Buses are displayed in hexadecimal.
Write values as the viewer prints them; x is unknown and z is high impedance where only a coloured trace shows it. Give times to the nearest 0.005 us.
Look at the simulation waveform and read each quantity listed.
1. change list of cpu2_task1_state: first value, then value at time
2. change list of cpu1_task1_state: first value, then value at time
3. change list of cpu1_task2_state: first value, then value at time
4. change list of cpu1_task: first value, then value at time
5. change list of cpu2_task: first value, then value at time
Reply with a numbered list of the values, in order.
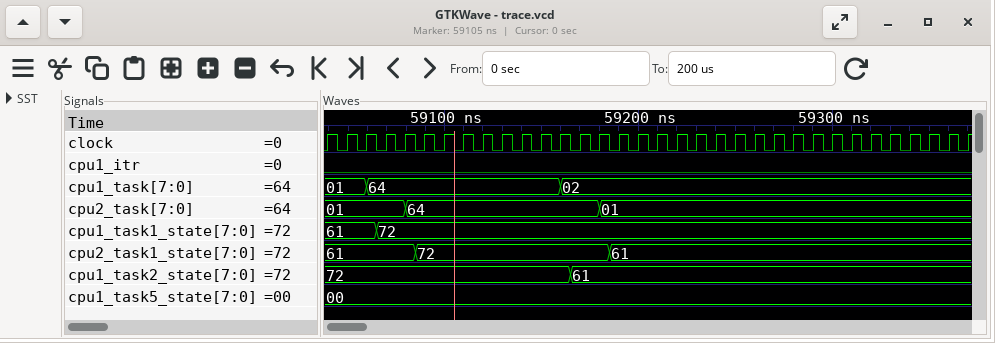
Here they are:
1. 61, 72 at 59.085 us, 61 at 59.185 us
2. 61, 72 at 59.065 us
3. 72, 61 at 59.165 us
4. 01, 64 at 59.06 us, 02 at 59.16 us
5. 01, 64 at 59.08 us, 01 at 59.18 us
